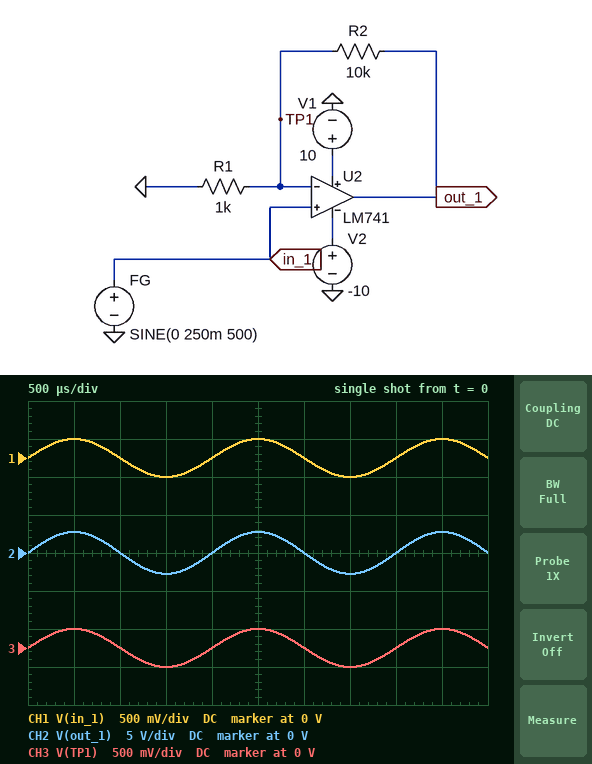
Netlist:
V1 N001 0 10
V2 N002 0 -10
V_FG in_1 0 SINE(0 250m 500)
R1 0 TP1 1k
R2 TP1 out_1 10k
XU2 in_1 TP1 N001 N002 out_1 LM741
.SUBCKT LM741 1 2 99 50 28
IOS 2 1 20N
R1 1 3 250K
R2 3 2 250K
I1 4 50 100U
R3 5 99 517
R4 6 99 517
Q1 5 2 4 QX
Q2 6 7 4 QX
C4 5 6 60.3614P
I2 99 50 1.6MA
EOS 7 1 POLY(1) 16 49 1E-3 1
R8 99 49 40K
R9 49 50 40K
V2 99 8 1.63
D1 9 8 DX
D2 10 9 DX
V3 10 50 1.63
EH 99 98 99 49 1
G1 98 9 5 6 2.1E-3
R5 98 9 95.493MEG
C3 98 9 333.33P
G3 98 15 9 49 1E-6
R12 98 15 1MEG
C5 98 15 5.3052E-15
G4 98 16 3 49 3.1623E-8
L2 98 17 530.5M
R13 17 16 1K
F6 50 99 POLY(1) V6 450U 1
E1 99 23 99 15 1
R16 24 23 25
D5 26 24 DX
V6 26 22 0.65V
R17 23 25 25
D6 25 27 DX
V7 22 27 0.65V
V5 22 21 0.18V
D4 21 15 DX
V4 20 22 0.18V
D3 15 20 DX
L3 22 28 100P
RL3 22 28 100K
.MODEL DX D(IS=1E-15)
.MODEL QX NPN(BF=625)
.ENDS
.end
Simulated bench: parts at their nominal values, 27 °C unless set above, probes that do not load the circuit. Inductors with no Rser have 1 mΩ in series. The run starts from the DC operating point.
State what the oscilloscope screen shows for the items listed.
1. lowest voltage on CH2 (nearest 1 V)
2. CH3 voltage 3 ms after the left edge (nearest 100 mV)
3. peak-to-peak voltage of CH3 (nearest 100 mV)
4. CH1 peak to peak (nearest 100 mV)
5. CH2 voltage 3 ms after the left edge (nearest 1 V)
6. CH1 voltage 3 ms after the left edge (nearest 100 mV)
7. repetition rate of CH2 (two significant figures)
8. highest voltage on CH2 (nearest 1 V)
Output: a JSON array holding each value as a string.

["-3 V", "0 V", "500 mV", "500 mV", "0 V", "0 V", "500 Hz", "3 V"]
